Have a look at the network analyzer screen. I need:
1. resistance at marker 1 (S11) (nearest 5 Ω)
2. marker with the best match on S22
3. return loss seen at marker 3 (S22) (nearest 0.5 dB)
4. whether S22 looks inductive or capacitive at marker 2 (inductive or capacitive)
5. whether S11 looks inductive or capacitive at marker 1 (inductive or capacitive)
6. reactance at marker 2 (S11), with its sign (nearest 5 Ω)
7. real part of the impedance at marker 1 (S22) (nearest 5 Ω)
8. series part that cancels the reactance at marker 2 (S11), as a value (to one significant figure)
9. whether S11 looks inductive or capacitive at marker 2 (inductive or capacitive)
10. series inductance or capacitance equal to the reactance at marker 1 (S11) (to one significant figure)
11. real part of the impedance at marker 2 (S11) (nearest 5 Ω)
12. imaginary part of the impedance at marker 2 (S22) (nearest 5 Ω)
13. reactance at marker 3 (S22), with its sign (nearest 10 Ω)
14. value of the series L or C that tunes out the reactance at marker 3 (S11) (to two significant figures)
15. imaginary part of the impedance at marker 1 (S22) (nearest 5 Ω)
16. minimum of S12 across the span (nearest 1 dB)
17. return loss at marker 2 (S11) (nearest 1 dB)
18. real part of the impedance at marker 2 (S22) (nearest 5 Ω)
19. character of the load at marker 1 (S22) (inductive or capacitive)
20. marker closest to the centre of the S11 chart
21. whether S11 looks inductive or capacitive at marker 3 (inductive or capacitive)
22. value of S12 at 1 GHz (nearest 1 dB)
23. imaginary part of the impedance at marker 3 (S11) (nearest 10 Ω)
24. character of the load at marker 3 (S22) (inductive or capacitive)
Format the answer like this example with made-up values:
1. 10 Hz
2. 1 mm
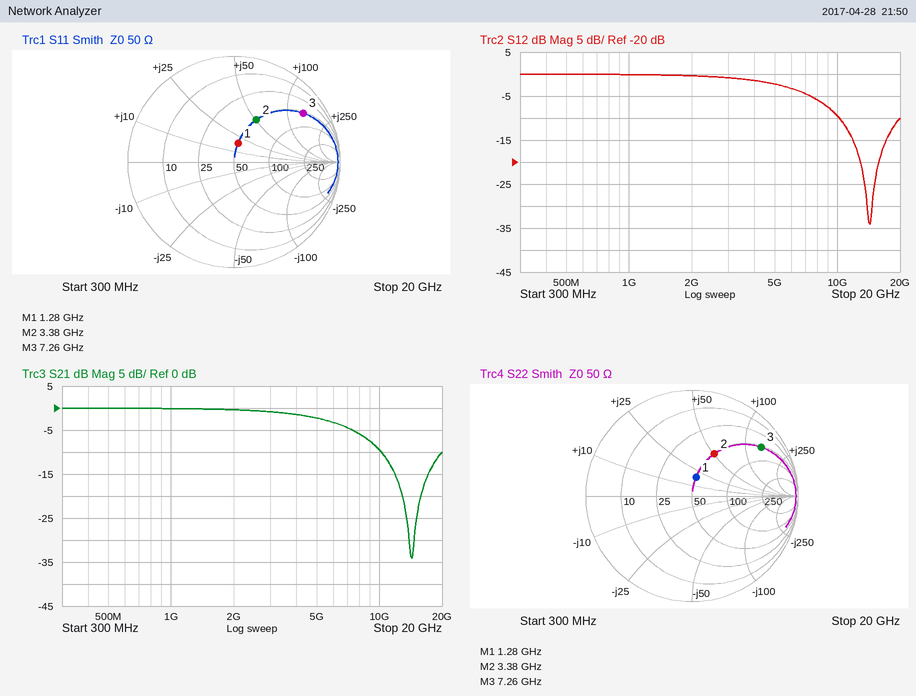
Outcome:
1. 50 Ω
2. marker 1
3. 2.0 dB
4. inductive
5. inductive
6. +50 Ω
7. 50 Ω
8. 900 fF
9. inductive
10. 2 nH
11. 50 Ω
12. +50 Ω
13. +140 Ω
14. 160 fF
15. +20 Ω
16. -34 dB
17. 7 dB
18. 50 Ω
19. inductive
20. marker 1
21. inductive
22. 0 dB
23. +140 Ω
24. inductive
